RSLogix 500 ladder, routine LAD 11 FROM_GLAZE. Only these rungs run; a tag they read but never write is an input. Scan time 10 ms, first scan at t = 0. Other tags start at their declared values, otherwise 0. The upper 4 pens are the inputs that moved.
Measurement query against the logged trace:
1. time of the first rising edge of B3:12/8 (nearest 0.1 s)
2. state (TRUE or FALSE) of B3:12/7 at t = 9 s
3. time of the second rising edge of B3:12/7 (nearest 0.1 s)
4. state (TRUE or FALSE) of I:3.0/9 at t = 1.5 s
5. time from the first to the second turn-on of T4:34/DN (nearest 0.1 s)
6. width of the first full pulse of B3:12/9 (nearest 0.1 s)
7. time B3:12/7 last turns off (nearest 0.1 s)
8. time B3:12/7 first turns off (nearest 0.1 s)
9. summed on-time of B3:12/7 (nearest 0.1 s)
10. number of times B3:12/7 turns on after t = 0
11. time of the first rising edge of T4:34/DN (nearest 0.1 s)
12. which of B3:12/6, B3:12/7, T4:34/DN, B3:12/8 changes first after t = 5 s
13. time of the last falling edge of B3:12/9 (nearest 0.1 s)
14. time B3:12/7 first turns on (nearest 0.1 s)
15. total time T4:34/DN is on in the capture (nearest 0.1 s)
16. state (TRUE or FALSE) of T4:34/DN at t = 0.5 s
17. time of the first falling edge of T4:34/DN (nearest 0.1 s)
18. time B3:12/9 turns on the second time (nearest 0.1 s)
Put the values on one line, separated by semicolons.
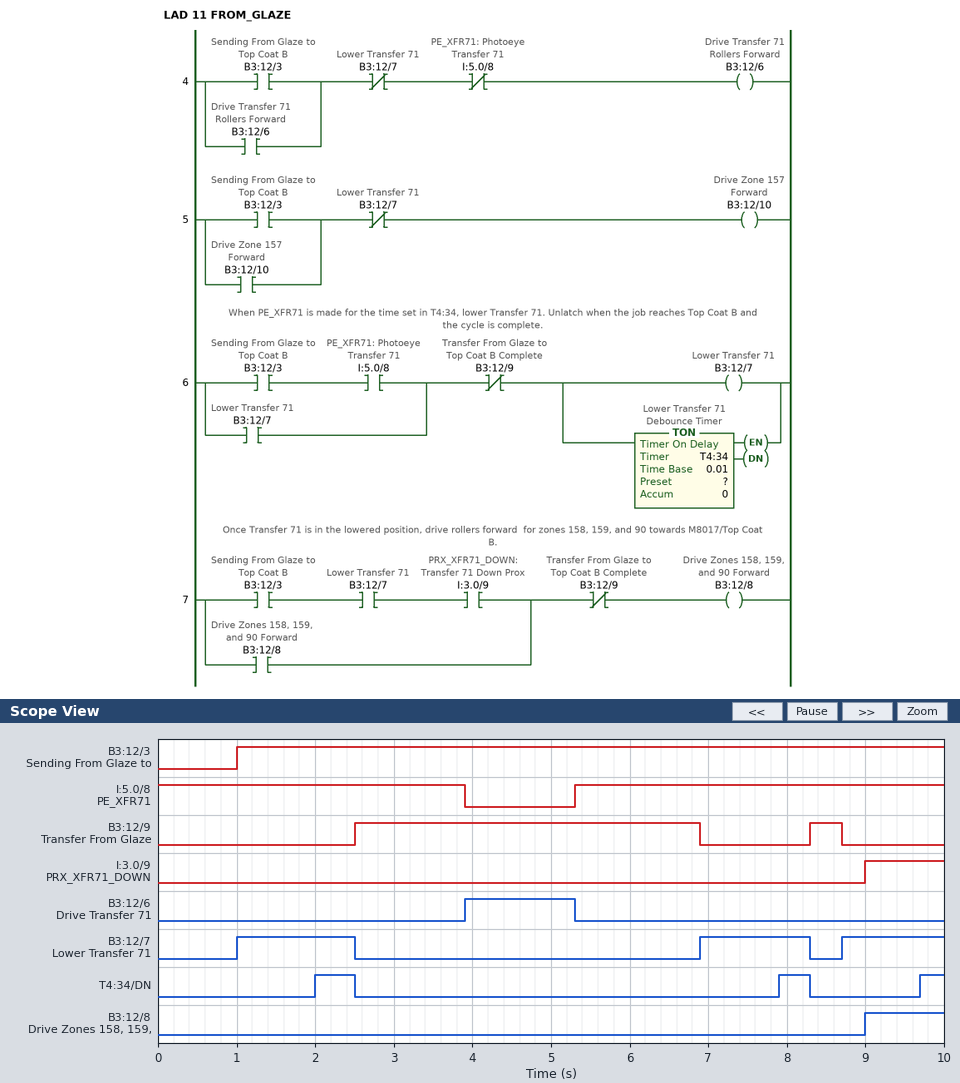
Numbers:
9.0 s; TRUE; 6.9 s; FALSE; 5.9 s; 4.4 s; 8.3 s; 2.5 s; 4.2 s; 3; 2.0 s; B3:12/6; 8.7 s; 1.0 s; 1.2 s; FALSE; 2.5 s; 8.3 s
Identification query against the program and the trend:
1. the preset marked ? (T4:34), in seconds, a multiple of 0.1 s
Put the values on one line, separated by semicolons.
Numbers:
1.0 s
